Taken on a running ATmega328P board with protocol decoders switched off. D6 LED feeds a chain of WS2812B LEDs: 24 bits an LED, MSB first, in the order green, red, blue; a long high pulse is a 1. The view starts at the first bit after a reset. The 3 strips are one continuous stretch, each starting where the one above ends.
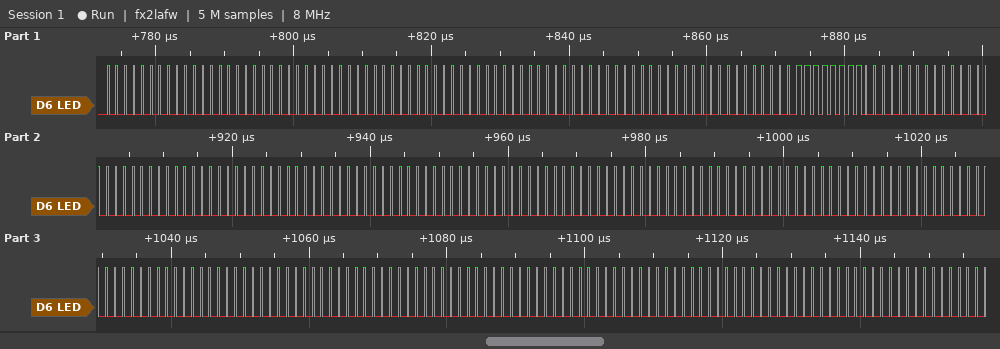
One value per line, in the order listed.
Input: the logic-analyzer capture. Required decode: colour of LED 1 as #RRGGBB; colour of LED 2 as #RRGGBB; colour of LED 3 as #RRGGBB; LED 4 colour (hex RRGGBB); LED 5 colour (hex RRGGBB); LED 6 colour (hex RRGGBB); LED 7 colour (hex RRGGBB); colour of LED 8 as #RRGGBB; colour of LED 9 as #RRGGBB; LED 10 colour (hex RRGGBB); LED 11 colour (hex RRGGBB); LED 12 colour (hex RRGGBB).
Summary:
#000000
#000000
#000000
#FF0000
#000000
#000000
#000000
#000000
#000000
#000000
#000000
#000000
